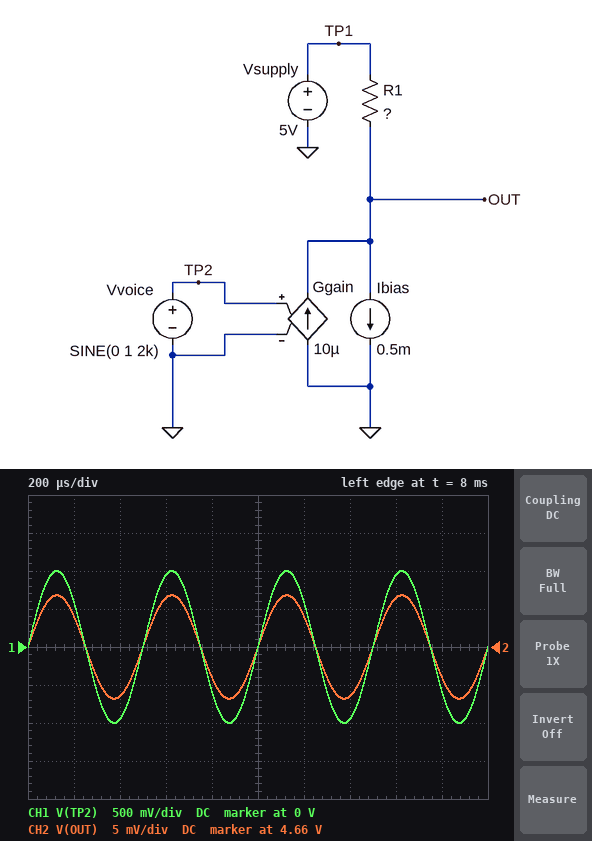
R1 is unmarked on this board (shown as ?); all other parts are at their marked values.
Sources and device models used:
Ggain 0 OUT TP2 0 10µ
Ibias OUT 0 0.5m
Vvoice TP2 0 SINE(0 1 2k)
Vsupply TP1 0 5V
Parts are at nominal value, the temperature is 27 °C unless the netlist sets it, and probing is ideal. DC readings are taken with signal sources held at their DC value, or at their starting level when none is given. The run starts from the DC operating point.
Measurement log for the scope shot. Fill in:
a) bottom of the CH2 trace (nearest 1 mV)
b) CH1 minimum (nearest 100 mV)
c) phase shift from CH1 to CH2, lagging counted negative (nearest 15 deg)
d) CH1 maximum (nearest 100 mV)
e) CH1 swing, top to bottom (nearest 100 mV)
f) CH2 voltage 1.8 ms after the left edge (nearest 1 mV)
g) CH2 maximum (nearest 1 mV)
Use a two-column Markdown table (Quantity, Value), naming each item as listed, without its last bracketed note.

| Quantity | Value |
|---|---|
| bottom of the CH2 trace | 4.653 V |
| CH1 minimum | -1.0 V |
| phase shift from CH1 to CH2, lagging counted negative | 0 deg |
| CH1 maximum | 1.0 V |
| CH1 swing, top to bottom | 2.0 V |
| CH2 voltage 1.8 ms after the left edge | 4.656 V |
| CH2 maximum | 4.667 V |
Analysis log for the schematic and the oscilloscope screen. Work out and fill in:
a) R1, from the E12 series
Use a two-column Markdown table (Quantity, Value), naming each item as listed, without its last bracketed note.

| Quantity | Value |
|---|---|
| R1, from the E12 series | 680 Ω |
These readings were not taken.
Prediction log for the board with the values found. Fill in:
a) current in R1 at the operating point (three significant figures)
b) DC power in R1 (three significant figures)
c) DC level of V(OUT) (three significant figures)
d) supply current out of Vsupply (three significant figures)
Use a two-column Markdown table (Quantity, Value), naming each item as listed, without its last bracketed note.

| Quantity | Value |
|---|---|
| current in R1 at the operating point | 500 µA |
| DC power in R1 | 170 µW |
| DC level of V(OUT) | 4.66 V |
| supply current out of Vsupply | 500 µA |
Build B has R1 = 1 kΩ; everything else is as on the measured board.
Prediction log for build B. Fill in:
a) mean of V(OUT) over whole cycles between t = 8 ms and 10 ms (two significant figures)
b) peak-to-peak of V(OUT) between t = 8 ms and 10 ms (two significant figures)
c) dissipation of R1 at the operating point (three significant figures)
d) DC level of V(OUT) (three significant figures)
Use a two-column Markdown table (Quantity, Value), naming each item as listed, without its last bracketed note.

| Quantity | Value |
|---|---|
| mean of V(OUT) over whole cycles between t = 8 ms and 10 ms | 4.5 V |
| peak-to-peak of V(OUT) between t = 8 ms and 10 ms | 20 mV |
| dissipation of R1 at the operating point | 250 µW |
| DC level of V(OUT) | 4.50 V |
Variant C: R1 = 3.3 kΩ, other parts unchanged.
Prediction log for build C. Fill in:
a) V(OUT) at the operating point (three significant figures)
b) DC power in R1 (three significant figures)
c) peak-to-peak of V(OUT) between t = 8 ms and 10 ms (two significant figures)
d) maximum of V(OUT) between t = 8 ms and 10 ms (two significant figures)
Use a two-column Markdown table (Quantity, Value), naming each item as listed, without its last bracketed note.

| Quantity | Value |
|---|---|
| V(OUT) at the operating point | 3.35 V |
| DC power in R1 | 825 µW |
| peak-to-peak of V(OUT) between t = 8 ms and 10 ms | 66 mV |
| maximum of V(OUT) between t = 8 ms and 10 ms | 3.4 V |
